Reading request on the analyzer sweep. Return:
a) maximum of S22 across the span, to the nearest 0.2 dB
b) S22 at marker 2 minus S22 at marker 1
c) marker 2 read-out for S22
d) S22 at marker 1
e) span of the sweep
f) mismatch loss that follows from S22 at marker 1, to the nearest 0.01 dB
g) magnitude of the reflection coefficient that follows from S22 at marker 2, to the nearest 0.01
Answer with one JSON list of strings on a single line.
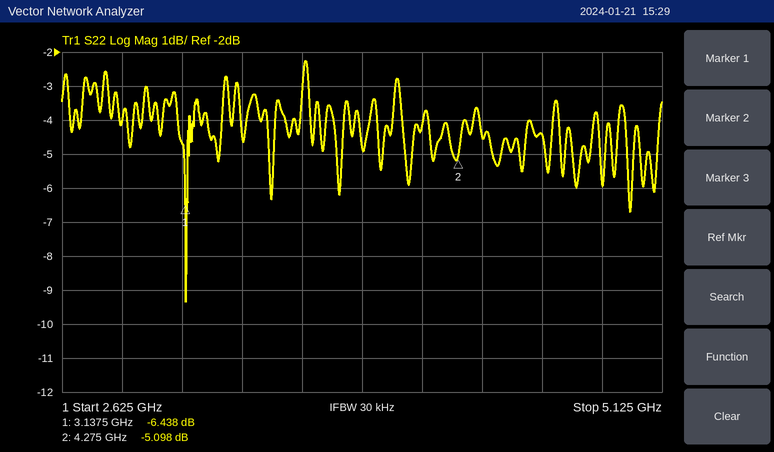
["-2.2 dB", "1.340 dB", "-5.098 dB", "-6.438 dB", "2.5 GHz", "1.12 dB", "0.56"]
